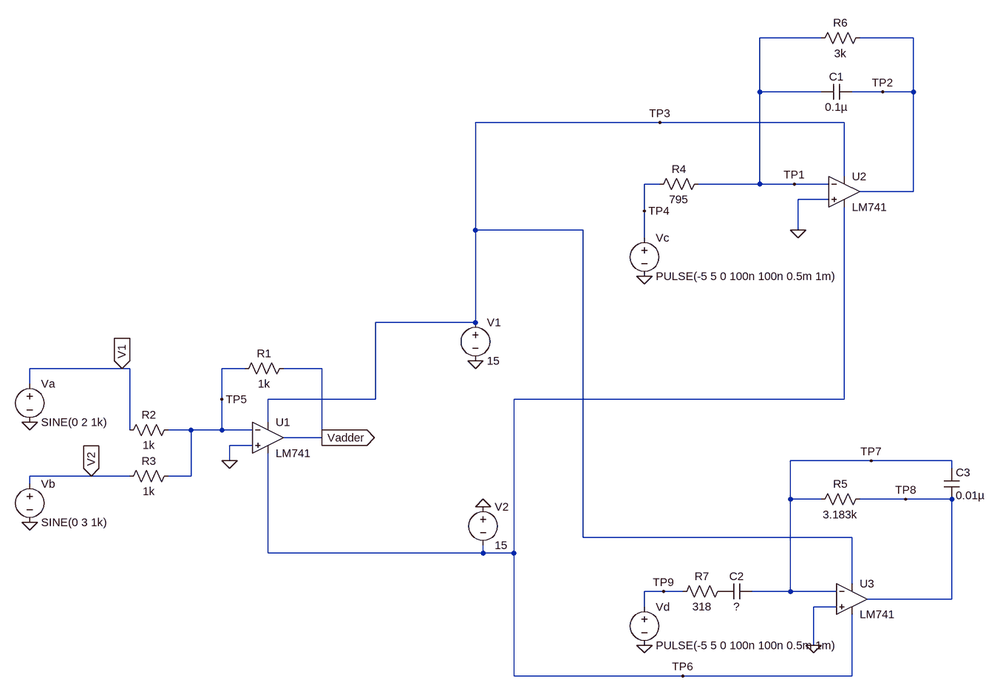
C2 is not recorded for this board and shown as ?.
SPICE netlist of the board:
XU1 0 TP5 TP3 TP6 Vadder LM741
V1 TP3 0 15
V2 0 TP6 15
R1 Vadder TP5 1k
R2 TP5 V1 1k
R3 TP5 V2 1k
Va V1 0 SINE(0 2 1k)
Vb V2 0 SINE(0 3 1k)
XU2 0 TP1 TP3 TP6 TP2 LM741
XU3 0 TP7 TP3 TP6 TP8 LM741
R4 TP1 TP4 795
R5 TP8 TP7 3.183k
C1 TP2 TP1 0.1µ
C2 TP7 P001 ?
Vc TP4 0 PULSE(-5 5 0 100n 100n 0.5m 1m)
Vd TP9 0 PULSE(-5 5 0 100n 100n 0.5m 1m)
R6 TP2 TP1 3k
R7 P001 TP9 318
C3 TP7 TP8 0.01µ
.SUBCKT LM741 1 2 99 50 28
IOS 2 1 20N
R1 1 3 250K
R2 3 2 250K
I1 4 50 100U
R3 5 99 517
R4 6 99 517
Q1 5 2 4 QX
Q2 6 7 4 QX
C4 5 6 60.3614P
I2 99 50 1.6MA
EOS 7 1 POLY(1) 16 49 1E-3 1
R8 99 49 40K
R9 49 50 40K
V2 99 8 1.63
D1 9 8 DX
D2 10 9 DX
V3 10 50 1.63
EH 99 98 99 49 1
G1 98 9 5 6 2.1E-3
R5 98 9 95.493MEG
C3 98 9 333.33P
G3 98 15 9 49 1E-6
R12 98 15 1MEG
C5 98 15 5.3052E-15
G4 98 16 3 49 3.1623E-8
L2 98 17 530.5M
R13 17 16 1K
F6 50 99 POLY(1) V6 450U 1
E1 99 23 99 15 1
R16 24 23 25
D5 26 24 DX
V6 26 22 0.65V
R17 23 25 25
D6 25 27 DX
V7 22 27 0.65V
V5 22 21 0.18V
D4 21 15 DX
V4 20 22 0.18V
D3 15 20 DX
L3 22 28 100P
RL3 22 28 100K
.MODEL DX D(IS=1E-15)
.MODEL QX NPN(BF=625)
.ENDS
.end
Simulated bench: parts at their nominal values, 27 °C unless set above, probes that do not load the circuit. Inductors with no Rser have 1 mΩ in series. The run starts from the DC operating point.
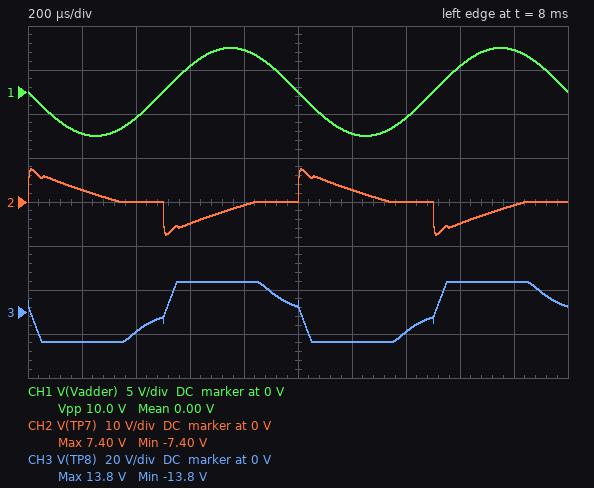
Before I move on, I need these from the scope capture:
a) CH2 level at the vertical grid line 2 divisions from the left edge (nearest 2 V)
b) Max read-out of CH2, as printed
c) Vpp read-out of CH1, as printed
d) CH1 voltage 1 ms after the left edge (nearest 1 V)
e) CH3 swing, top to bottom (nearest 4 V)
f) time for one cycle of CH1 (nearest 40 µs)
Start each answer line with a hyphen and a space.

- 0 V
- 7.40 V
- 10.0 V
- 0 V
- 28 V
- 1.00 ms
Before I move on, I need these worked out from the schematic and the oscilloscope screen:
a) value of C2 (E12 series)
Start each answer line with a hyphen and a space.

- 220 nF
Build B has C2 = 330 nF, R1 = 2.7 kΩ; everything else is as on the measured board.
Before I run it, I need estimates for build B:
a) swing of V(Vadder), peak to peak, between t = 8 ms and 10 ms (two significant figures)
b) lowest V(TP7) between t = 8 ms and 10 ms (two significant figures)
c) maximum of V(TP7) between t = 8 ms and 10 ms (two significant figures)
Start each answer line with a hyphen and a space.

- 27 V
- -7.7 V
- 7.7 V
